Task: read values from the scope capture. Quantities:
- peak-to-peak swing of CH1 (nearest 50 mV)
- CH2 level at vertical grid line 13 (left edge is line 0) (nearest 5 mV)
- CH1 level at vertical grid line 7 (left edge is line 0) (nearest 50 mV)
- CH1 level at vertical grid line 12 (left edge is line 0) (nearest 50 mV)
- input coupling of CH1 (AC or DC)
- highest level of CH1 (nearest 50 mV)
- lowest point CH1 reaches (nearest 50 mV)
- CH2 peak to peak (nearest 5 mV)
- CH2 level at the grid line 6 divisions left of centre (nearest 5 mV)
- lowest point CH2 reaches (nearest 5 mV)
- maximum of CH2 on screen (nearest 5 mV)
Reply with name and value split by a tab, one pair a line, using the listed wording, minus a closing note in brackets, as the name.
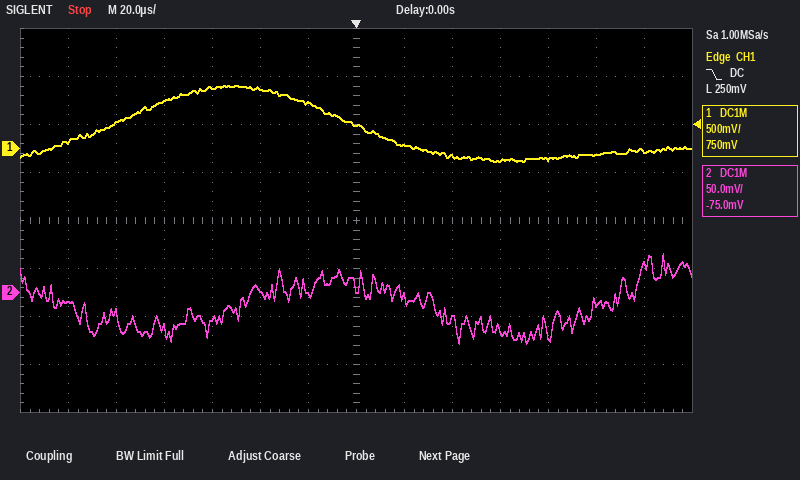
peak-to-peak swing of CH1	800 mV
CH2 level at vertical grid line 13 (left edge is line 0)	30 mV
CH1 level at vertical grid line 7 (left edge is line 0)	250 mV
CH1 level at vertical grid line 12 (left edge is line 0)	-50 mV
input coupling of CH1	DC
highest level of CH1	650 mV
lowest point CH1 reaches	-150 mV
CH2 peak to peak	95 mV
CH2 level at the grid line 6 divisions left of centre	-10 mV
lowest point CH2 reaches	-55 mV
maximum of CH2 on screen	40 mV
